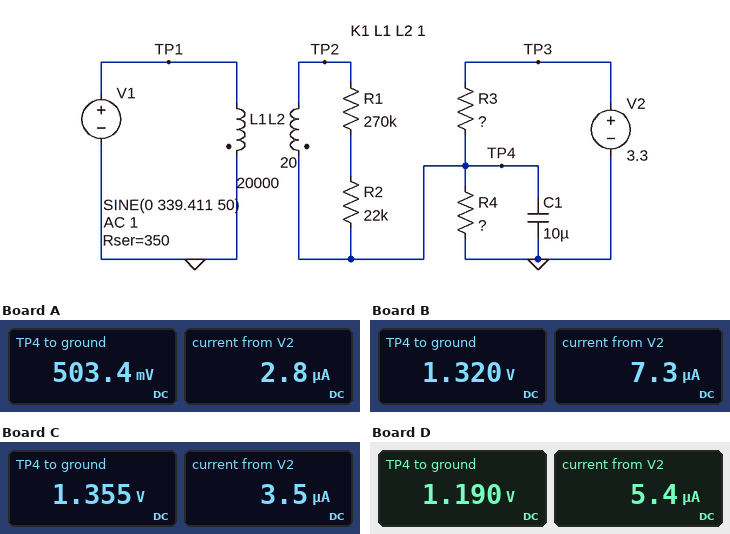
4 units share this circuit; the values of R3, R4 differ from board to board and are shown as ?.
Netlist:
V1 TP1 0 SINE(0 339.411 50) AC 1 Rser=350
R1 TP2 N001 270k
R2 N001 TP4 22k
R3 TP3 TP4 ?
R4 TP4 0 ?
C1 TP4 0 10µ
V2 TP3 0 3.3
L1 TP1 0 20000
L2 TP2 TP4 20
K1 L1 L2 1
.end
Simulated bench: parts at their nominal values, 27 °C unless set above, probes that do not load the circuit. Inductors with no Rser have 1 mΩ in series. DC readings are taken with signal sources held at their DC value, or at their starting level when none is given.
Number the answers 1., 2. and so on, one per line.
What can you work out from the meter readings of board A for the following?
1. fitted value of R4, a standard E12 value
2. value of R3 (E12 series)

1. 180 kΩ
2. 1 MΩ
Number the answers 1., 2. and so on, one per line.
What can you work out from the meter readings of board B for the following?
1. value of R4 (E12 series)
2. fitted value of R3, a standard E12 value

1. 180 kΩ
2. 270 kΩ
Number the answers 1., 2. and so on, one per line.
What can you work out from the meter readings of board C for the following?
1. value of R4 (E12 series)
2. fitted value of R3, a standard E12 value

1. 390 kΩ
2. 560 kΩ
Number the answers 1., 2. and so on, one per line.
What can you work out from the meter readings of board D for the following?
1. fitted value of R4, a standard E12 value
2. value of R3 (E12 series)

1. 220 kΩ
2. 390 kΩ
